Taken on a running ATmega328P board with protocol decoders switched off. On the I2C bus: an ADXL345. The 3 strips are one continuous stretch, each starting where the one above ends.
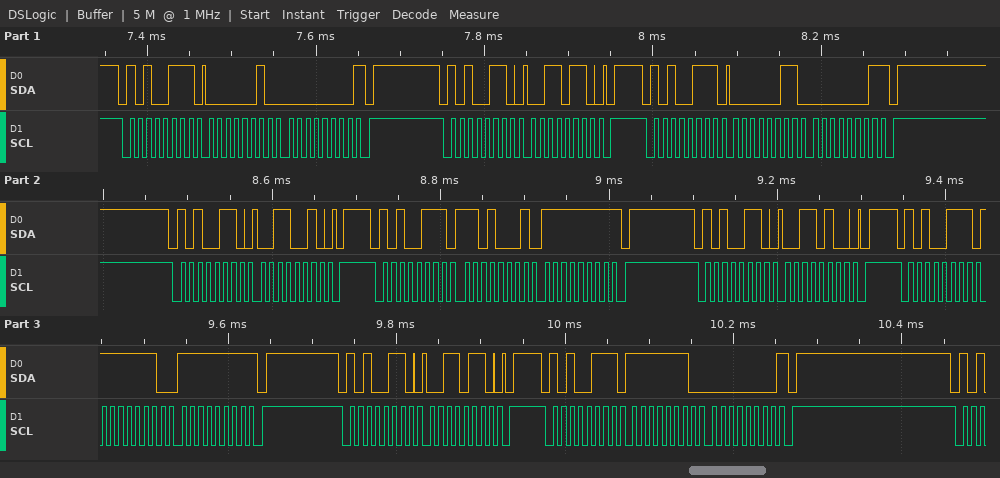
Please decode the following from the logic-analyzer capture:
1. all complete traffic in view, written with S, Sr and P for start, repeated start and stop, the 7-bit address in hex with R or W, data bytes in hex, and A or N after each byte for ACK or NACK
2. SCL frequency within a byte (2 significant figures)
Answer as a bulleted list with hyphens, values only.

- S 53R A 02 A 00 N P S 53W A 36 A P S 53R A 03 A 01 N P S 53W A 32 A P S 53R A D1 A FF N P S 53W A 34 A P S 53R A FE A FF N P S 53W A 36 A P S 53R A FE A 00 N P
- 100 kHz
